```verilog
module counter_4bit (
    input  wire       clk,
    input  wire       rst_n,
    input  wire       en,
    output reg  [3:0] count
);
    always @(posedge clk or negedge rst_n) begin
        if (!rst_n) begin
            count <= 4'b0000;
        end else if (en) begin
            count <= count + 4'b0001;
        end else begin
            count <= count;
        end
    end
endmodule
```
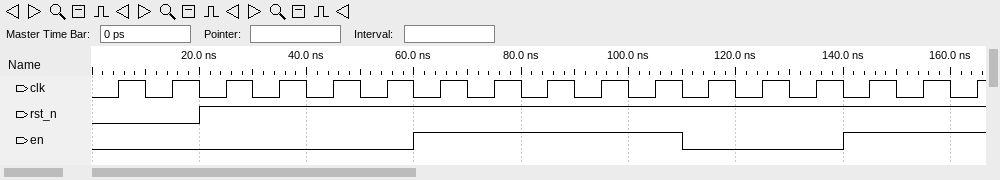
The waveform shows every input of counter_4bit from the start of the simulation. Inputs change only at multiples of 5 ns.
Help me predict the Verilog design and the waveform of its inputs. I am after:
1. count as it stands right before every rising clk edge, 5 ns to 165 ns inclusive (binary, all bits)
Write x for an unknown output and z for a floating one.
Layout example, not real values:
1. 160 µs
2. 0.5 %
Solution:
1. 0000, 0000, 0000, 0000, 0000, 0000, 0000, 0001, 0010, 0011, 0100, 0101, 0101, 0101, 0101, 0110, 0111
